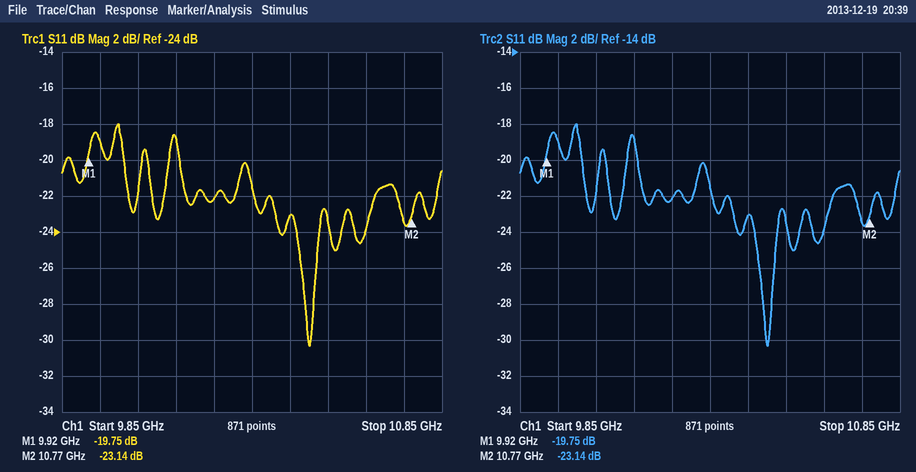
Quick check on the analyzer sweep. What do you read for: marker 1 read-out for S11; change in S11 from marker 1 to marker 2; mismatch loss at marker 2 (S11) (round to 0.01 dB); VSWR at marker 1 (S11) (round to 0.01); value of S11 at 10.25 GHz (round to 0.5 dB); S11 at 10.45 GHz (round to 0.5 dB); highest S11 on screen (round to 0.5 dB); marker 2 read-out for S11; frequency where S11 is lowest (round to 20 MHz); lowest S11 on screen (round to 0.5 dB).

-19.75 dB
-3.39 dB
0.02 dB
1.23
-22.0 dB
-23.0 dB
-18.0 dB
-23.14 dB
10.50 GHz
-30.5 dB
